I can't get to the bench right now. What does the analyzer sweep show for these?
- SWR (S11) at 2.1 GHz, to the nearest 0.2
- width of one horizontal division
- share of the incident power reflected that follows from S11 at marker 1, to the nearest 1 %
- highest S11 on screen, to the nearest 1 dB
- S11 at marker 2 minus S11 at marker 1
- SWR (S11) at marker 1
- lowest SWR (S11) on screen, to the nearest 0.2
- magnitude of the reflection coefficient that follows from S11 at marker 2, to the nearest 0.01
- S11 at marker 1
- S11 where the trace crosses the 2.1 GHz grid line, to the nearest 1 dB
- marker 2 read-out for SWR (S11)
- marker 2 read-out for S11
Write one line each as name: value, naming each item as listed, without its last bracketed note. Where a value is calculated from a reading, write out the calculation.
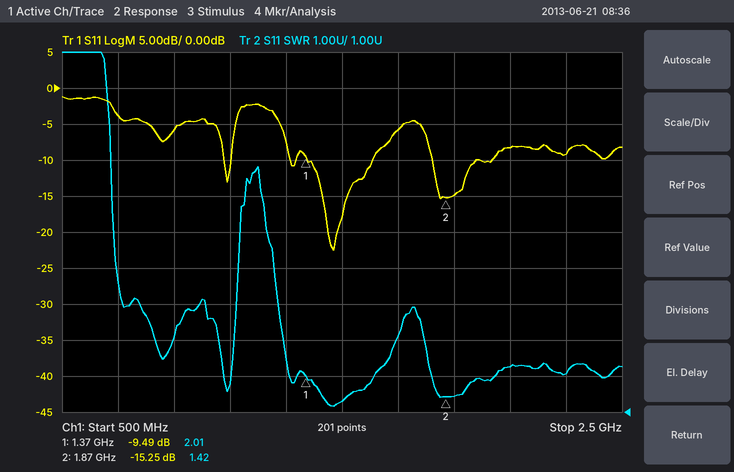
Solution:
SWR (S11) at 2.1 GHz, to the nearest 0.2: 2.2
width of one horizontal division: 200 MHz
share of the incident power reflected that follows from S11 at marker 1, to the nearest 1 %: 10^(-9.49/10) ≈ 11 %
highest S11 on screen, to the nearest 1 dB: -1 dB
S11 at marker 2 minus S11 at marker 1: -15.25 − (-9.49) = -5.76 dB
SWR (S11) at marker 1: 2.01
lowest SWR (S11) on screen, to the nearest 0.2: 1.2
magnitude of the reflection coefficient that follows from S11 at marker 2, to the nearest 0.01: 10^(-15.25/20) ≈ 0.17
S11 at marker 1: -9.49 dB
S11 where the trace crosses the 2.1 GHz grid line, to the nearest 1 dB: -8 dB
marker 2 read-out for SWR: 1.42
marker 2 read-out for S11: -15.25 dB
